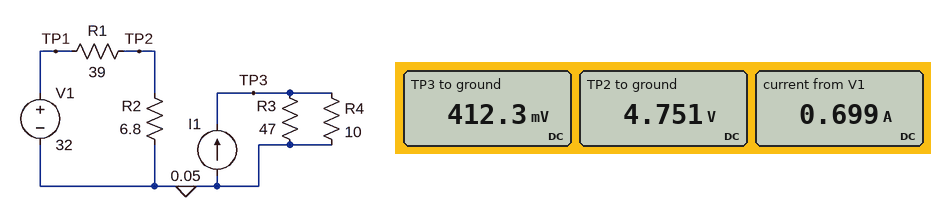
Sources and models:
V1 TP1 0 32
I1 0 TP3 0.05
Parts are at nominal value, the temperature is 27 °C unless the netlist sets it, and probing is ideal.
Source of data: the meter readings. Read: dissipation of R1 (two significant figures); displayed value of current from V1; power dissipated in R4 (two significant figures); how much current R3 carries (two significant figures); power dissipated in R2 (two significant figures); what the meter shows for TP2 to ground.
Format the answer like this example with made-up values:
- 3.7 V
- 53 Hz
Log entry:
- 19 W
- 0.699 A
- 17 mW
- 8.8 mA
- 3.3 W
- 4.751 V
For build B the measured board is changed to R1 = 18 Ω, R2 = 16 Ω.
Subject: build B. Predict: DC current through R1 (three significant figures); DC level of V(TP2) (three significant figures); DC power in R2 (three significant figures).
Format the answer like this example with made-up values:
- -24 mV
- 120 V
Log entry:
- 941 mA
- 15.1 V
- 14.2 W
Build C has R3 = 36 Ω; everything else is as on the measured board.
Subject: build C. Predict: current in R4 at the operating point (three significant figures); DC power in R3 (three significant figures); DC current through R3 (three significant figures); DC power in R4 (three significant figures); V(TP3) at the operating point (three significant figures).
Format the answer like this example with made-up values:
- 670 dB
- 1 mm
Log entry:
- 39.1 mA
- 4.25 mW
- 10.9 mA
- 15.3 mW
- 391 mV
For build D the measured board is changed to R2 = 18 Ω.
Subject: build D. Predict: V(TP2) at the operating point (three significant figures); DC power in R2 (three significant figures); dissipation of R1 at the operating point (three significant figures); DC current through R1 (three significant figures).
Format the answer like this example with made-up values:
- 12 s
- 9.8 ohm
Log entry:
- 10.1 V
- 5.67 W
- 12.3 W
- 561 mA
